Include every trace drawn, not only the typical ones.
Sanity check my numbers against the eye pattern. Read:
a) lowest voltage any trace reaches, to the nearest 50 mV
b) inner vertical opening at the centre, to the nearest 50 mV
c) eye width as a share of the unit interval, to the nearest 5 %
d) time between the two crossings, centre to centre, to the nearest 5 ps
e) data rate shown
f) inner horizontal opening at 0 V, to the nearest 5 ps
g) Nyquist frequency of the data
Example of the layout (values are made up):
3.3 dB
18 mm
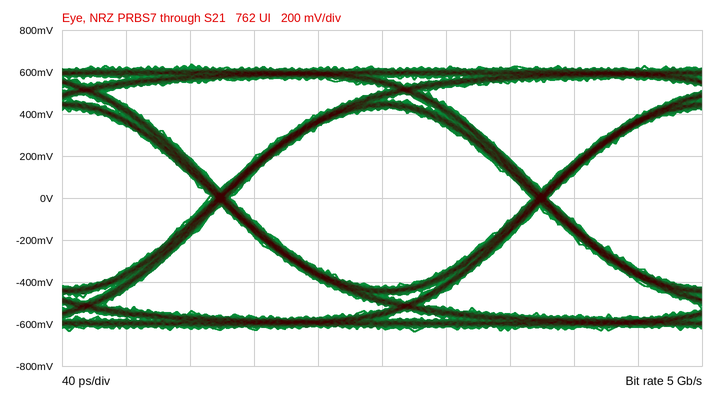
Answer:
-650 mV
850 mV
95 %
200 ps
5 Gb/s
190 ps
2.5 GHz
